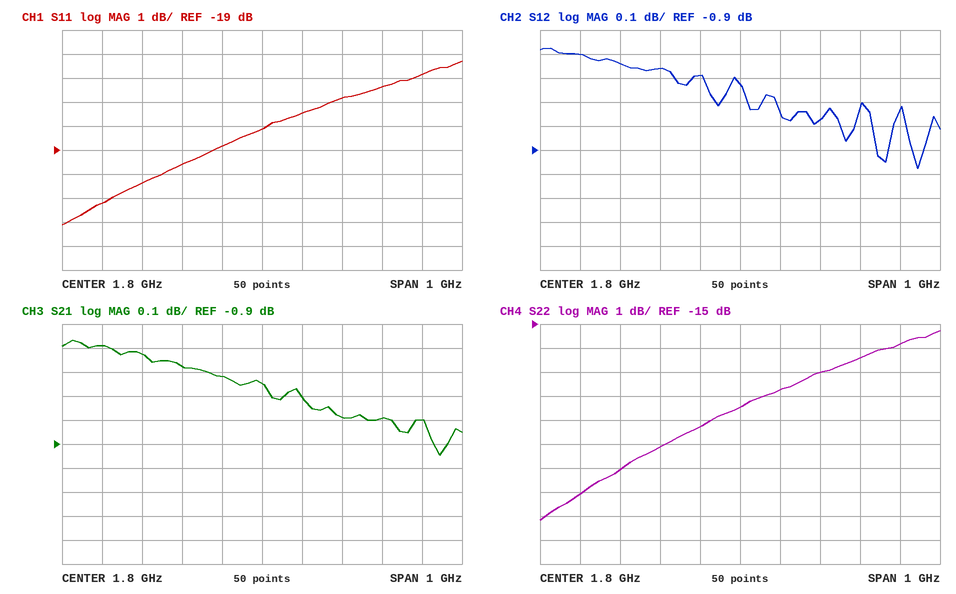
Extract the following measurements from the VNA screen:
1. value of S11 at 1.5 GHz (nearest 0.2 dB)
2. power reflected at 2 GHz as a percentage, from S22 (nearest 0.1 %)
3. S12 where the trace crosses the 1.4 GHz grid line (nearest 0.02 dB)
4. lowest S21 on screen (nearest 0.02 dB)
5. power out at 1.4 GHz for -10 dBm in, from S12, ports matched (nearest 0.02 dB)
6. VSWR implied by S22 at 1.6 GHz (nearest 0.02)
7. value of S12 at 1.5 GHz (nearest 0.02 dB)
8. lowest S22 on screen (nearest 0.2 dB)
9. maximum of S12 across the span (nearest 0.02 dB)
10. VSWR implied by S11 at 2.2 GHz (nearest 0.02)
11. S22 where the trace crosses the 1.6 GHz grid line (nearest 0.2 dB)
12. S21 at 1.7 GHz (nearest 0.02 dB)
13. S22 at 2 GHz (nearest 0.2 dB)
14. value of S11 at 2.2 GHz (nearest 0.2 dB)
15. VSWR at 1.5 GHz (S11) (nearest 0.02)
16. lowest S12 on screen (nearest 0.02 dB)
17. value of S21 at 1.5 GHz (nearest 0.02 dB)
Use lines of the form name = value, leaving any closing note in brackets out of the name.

value of S11 at 1.5 GHz = -20.4 dB
power reflected at 2 GHz as a percentage, from S22 = 2.0 %
S12 where the trace crosses the 1.4 GHz grid line = -0.50 dB
lowest S21 on screen = -0.94 dB
power out at 1.4 GHz for -10 dBm in, from S12, ports matched = -10.50 dBm
VSWR implied by S22 at 1.6 GHz = 1.22
value of S12 at 1.5 GHz = -0.54 dB
lowest S22 on screen = -23.2 dB
maximum of S12 across the span = -0.48 dB
VSWR implied by S11 at 2.2 GHz = 1.38
S22 where the trace crosses the 1.6 GHz grid line = -20.2 dB
S21 at 1.7 GHz = -0.62 dB
S22 at 2 GHz = -17.0 dB
value of S11 at 2.2 GHz = -15.8 dB
VSWR at 1.5 GHz (S11) = 1.22
lowest S12 on screen = -0.98 dB
value of S21 at 1.5 GHz = -0.52 dB
